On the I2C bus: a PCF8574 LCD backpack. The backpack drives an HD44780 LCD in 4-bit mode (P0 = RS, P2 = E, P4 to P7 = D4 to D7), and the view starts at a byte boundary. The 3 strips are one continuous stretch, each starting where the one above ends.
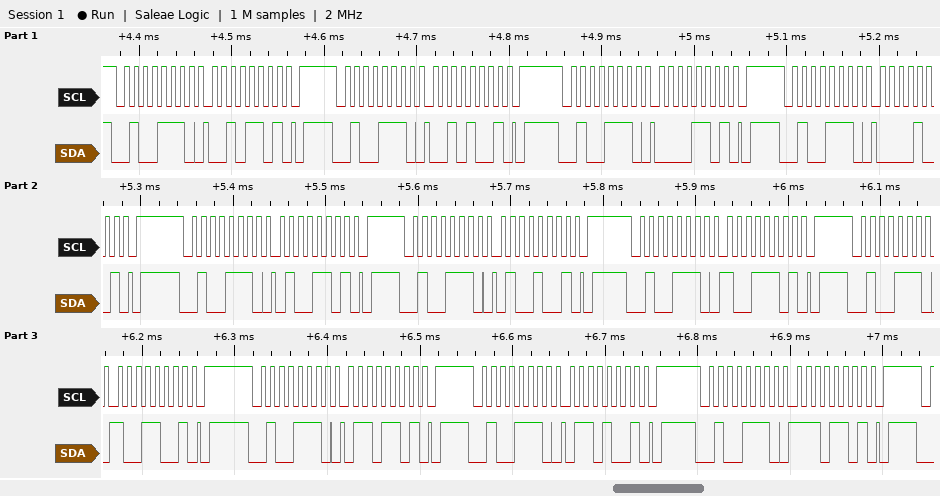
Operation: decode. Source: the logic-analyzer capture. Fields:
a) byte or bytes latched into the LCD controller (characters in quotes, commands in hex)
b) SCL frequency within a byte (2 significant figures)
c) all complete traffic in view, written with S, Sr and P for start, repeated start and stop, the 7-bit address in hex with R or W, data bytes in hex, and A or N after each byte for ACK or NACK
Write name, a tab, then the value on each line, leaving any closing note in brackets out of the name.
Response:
byte or bytes latched into the LCD controller	' ' 'I'
SCL frequency within a byte	100 kHz
all complete traffic in view, written with S, Sr and P for start, repeated start and stop, the 7-bit address in hex with R or W, data bytes in hex, and A or N after each byte for ACK or NACK	S 27W A 2D A P S 27W A 29 A P S 27W A 0D A P S 27W A 09 A P S 27W A 4D A P S 27W A 49 A P S 27W A 9D A P S 27W A 99 A P S 27W A 6D A P S 27W A 69 A P S 27W A ED A P
